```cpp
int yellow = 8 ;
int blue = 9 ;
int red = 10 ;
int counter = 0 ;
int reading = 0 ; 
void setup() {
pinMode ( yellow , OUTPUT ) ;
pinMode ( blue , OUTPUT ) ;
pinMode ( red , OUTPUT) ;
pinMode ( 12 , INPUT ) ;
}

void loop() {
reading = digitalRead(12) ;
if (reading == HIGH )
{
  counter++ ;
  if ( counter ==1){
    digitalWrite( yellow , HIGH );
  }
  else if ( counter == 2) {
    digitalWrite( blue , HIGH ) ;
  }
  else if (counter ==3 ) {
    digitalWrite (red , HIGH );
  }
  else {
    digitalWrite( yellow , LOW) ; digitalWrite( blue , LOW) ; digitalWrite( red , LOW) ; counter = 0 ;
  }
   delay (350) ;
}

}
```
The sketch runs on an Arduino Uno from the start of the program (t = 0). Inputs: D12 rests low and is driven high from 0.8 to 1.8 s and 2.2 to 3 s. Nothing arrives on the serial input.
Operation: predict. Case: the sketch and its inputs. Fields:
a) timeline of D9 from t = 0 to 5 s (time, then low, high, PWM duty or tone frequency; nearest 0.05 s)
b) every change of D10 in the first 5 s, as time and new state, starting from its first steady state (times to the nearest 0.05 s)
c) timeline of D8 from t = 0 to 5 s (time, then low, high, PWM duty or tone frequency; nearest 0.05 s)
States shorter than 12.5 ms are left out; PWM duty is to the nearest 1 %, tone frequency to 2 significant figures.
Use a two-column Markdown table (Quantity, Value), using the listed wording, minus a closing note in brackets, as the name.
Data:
| Quantity | Value |
|---|---|
| timeline of D9 from t = 0 to 5 s | 0 s low; 1.15 s high; 2.2 s low; 2.9 s high |
| every change of D10 in the first 5 s, as time and new state, starting from its first steady state | 0 s low; 1.5 s high; 2.2 s low |
| timeline of D8 from t = 0 to 5 s | 0 s low; 0.8 s high; 2.2 s low; 2.55 s high |
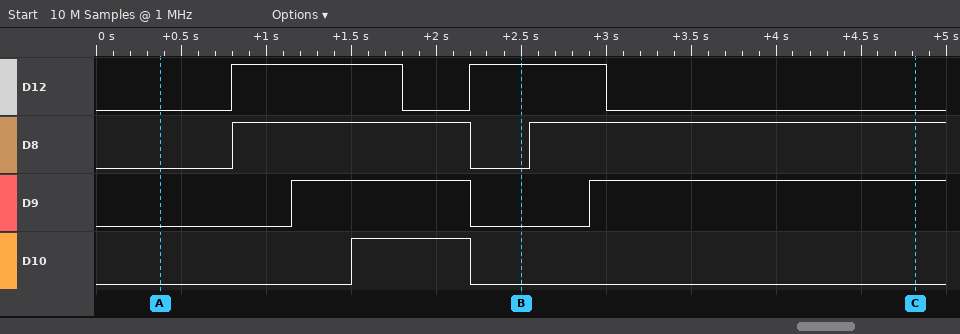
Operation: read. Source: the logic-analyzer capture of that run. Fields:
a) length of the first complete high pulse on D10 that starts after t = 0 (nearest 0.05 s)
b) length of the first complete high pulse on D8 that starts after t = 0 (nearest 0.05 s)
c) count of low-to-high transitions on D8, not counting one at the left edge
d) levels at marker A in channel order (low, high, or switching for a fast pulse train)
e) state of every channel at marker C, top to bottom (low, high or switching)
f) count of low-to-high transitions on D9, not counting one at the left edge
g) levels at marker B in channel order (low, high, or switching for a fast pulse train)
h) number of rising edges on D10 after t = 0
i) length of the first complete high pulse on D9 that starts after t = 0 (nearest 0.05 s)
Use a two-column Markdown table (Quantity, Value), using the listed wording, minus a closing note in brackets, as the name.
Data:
| Quantity | Value |
|---|---|
| length of the first complete high pulse on D10 that starts after t = 0 | 0.70 s |
| length of the first complete high pulse on D8 that starts after t = 0 | 1.40 s |
| count of low-to-high transitions on D8, not counting one at the left edge | 2 |
| levels at marker A in channel order | D12 low, D8 low, D9 low, D10 low |
| state of every channel at marker C, top to bottom | D12 low, D8 high, D9 high, D10 low |
| count of low-to-high transitions on D9, not counting one at the left edge | 2 |
| levels at marker B in channel order | D12 high, D8 low, D9 low, D10 low |
| number of rising edges on D10 after t = 0 | 1 |
| length of the first complete high pulse on D9 that starts after t = 0 | 1.05 s |
